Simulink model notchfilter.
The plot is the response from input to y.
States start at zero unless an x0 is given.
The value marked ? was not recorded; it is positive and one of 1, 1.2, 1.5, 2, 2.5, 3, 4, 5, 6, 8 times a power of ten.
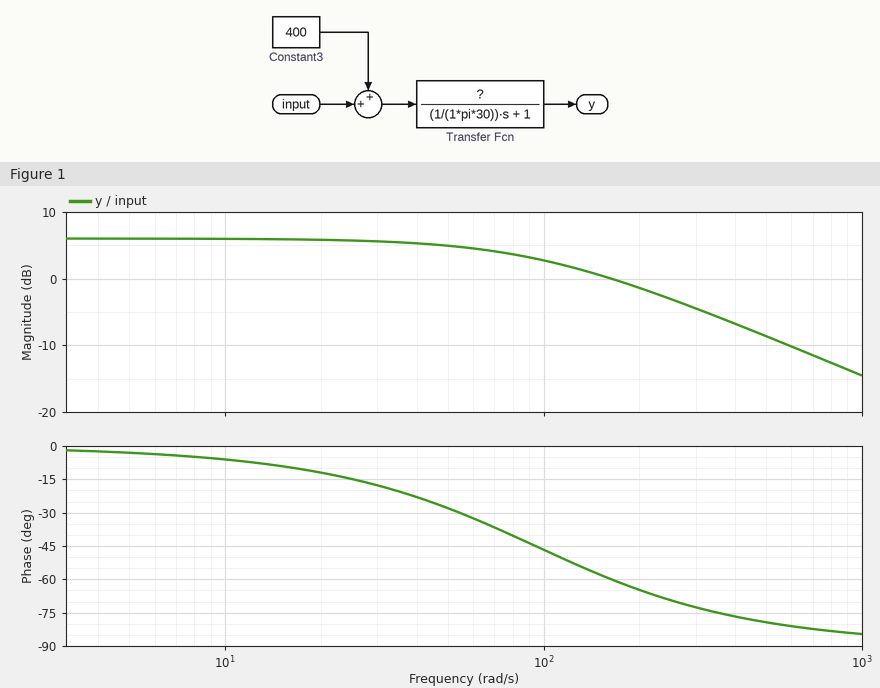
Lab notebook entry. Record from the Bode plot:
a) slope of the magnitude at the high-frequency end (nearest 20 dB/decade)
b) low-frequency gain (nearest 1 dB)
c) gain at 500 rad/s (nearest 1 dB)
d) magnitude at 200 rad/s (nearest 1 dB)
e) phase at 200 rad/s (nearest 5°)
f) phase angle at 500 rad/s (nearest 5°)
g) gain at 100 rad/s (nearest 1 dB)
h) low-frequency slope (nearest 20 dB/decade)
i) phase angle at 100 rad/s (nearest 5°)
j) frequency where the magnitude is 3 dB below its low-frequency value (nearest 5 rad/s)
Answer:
-20 dB/decade
6 dB
-9 dB
-1 dB
-65°
-80°
3 dB
0 dB/decade
-45°
95 rad/s
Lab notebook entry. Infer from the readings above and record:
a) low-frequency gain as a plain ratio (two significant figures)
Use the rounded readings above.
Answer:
2.0
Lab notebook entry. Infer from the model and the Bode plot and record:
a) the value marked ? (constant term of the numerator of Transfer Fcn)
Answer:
2
